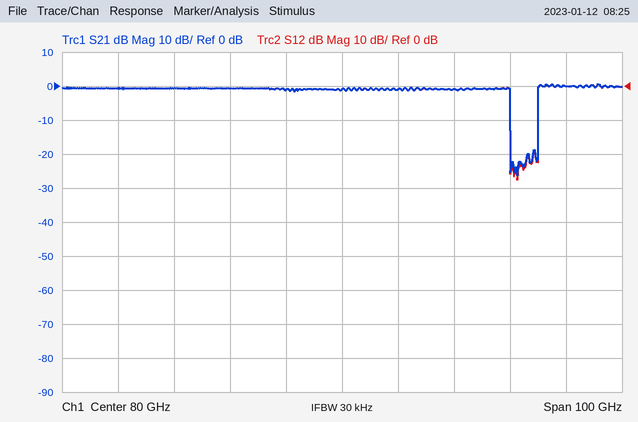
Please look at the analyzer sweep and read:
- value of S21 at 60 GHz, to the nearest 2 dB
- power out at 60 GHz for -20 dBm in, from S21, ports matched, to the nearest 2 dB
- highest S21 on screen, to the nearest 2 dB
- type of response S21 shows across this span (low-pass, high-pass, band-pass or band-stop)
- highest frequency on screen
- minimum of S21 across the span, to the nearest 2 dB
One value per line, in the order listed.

0 dB
-20 dBm
0 dB
band-stop
130 GHz
-26 dB
